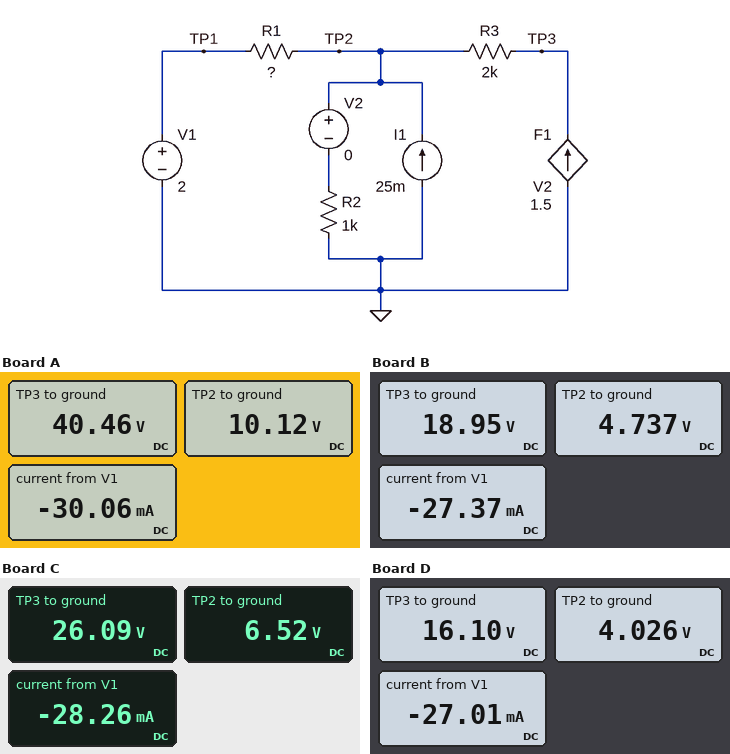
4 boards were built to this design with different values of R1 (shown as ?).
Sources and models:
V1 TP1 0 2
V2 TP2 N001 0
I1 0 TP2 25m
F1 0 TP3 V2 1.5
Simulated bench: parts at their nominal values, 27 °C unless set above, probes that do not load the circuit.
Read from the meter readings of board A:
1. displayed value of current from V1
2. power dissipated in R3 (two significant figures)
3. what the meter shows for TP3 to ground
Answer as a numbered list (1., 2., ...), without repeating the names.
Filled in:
1. -30.06 mA
2. 460 mW
3. 40.46 V
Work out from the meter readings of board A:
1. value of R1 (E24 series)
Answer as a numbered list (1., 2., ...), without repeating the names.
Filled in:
1. 270 Ω
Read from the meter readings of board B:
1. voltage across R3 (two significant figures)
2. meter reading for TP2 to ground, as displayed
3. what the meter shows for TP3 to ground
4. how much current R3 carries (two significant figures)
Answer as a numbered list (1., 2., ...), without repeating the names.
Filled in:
1. 14 V
2. 4.737 V
3. 18.95 V
4. 7.1 mA
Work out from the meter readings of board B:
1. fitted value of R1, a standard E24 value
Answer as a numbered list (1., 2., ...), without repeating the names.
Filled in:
1. 100 Ω
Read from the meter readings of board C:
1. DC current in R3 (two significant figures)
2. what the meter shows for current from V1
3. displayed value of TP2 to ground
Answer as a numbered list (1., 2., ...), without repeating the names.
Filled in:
1. 9.8 mA
2. -28.26 mA
3. 6.52 V
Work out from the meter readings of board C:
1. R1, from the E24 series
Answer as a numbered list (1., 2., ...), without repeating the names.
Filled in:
1. 160 Ω
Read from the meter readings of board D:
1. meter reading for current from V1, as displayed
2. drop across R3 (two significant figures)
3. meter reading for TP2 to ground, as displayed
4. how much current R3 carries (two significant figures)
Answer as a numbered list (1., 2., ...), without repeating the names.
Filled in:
1. -27.01 mA
2. 12 V
3. 4.026 V
4. 6.0 mA
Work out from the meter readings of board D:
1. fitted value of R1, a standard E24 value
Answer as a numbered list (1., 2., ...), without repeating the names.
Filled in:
1. 75 Ω
